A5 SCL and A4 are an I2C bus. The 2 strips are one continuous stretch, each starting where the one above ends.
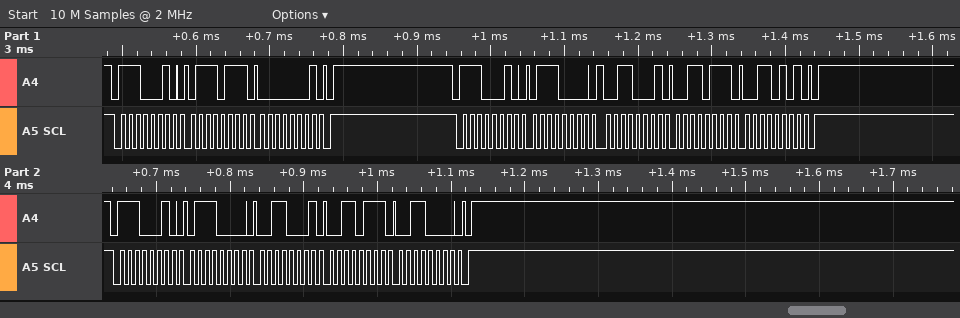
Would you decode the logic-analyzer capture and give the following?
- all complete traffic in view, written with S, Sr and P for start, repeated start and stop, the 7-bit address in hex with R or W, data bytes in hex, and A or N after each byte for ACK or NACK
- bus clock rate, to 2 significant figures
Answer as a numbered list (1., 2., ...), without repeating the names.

1. S 71W A 77 A 01 A P S 71W A 70 A 31 A 37 A 35 A P S 71W A 70 A 31 A 37 A 30 A P
2. 100 kHz
